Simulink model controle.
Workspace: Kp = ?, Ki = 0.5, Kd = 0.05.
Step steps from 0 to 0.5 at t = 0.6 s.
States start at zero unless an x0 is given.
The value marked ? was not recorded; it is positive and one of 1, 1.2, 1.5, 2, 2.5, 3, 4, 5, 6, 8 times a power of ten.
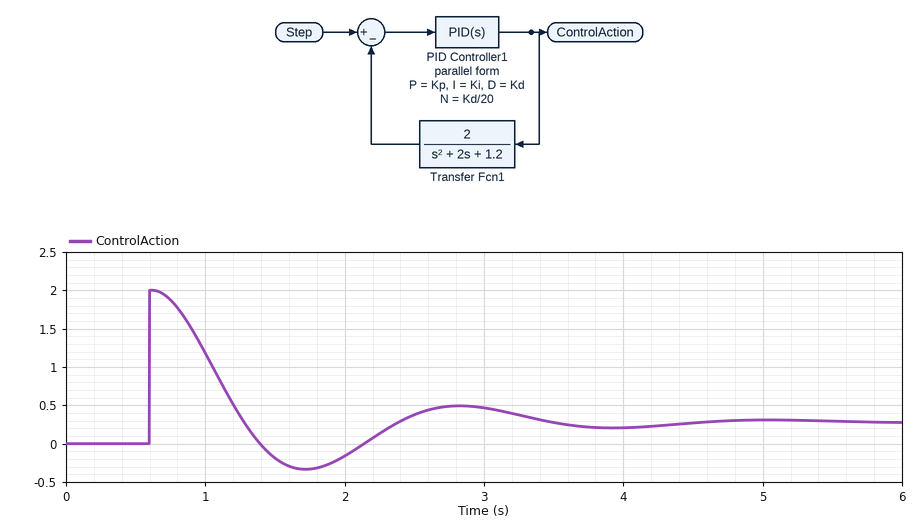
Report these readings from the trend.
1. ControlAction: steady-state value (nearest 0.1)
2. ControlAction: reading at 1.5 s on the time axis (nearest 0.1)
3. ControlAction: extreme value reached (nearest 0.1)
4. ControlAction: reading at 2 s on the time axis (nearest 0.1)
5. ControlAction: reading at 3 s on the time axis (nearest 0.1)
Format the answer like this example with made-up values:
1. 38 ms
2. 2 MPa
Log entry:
1. 0.3
2. -0.2
3. 2.0
4. -0.2
5. 0.5
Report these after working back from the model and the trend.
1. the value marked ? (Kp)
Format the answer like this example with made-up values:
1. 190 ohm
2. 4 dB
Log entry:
1. 4
